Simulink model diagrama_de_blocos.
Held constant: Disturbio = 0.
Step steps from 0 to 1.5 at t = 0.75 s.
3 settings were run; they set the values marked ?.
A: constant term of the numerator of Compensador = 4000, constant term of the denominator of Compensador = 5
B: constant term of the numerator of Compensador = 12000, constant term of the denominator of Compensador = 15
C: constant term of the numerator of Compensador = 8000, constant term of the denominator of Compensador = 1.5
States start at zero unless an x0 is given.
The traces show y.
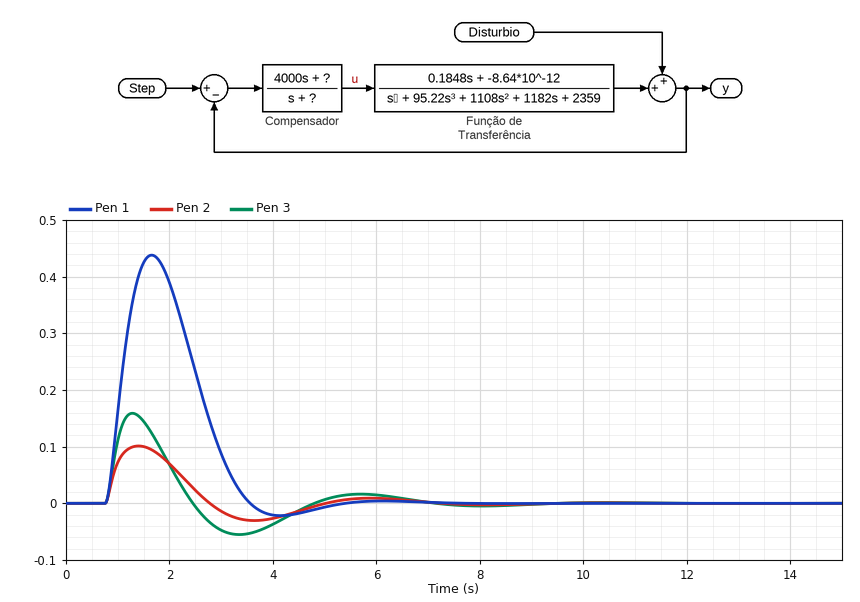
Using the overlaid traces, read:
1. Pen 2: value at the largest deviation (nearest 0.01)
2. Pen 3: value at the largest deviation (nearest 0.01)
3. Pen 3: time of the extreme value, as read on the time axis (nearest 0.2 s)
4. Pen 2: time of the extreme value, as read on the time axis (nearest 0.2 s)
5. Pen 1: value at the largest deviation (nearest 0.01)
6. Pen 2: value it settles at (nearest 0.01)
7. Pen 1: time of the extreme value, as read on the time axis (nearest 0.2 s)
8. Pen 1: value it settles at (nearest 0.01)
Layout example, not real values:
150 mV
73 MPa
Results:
0.10
0.16
1.2 s
1.4 s
0.44
0.00
1.6 s
0.00
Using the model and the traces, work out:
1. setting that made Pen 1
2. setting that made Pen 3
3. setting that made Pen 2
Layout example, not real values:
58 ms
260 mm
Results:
C
A
B
